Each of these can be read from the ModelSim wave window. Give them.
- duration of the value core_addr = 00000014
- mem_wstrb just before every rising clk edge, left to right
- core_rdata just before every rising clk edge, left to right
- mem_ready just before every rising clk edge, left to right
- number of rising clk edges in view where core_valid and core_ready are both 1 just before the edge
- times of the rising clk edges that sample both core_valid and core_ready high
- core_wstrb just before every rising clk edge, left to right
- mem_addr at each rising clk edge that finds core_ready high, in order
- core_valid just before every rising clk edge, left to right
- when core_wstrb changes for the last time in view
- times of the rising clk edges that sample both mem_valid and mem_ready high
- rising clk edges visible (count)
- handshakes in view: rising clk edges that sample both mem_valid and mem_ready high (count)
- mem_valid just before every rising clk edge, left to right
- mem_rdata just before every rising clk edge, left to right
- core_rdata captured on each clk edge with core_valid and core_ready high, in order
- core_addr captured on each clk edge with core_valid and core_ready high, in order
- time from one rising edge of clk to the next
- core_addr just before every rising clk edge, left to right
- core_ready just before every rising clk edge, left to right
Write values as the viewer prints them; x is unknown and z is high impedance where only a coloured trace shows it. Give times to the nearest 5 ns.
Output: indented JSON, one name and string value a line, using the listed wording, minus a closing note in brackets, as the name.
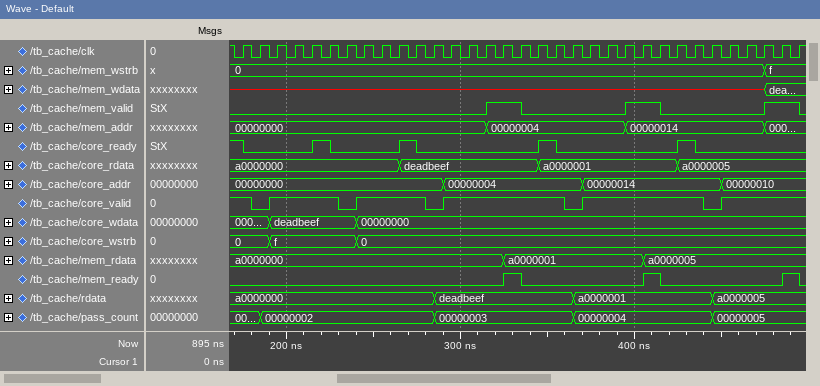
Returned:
{
  "duration of the value core_addr = 00000014": "80 ns",
  "mem_wstrb just before every rising clk edge, left to right": "0, 0, 0, 0, 0, 0, 0, 0, 0, 0, 0, 0, 0, 0, 0, 0, 0, 0, 0, 0, 0, 0, 0, 0, 0, 0, 0, 0, 0, 0, 0, f, f",
  "core_rdata just before every rising clk edge, left to right": "a0000000, a0000000, a0000000, a0000000, a0000000, a0000000, a0000000, a0000000, a0000000, a0000000, deadbeef, deadbeef, deadbeef, deadbeef, deadbeef, deadbeef, deadbeef, deadbeef, a0000001, a0000001, a0000001, a0000001, a0000001, a0000001, a0000001, a0000001, a0000005, a0000005, a0000005, a0000005, a0000005, a0000005, a0000005",
  "mem_ready just before every rising clk edge, left to right": "0 0 0 0 0 0 0 0 0 0 0 0 0 0 0 0 1 0 0 0 0 0 0 0 1 0 0 0 0 0 0 0 1",
  "number of rising clk edges in view where core_valid and core_ready are both 1 just before the edge": "5",
  "times of the rising clk edges that sample both core_valid and core_ready high": "175 ns, 225 ns, 275 ns, 355 ns, 435 ns",
  "core_wstrb just before every rising clk edge, left to right": "0, 0, f, f, f, f, f, 0, 0, 0, 0, 0, 0, 0, 0, 0, 0, 0, 0, 0, 0, 0, 0, 0, 0, 0, 0, 0, 0, 0, 0, 0, 0",
  "mem_addr at each rising clk edge that finds core_ready high, in order": "00000000, 00000000, 00000000, 00000004, 00000014",
  "core_valid just before every rising clk edge, left to right": "1 0 1 1 1 1 0 1 1 1 1 0 1 1 1 1 1 1 1 0 1 1 1 1 1 1 1 0 1 1 1 1 1",
  "when core_wstrb changes for the last time in view": "240 ns",
  "times of the rising clk edges that sample both mem_valid and mem_ready high": "335 ns, 415 ns, 495 ns",
  "rising clk edges visible": "33",
  "handshakes in view: rising clk edges that sample both mem_valid and mem_ready high": "3",
  "mem_valid just before every rising clk edge, left to right": "0 0 0 0 0 0 0 0 0 0 0 0 0 0 0 1 1 0 0 0 0 0 0 1 1 0 0 0 0 0 0 1 1",
  "mem_rdata just before every rising clk edge, left to right": "a0000000, a0000000, a0000000, a0000000, a0000000, a0000000, a0000000, a0000000, a0000000, a0000000, a0000000, a0000000, a0000000, a0000000, a0000000, a0000000, a0000001, a0000001, a0000001, a0000001, a0000001, a0000001, a0000001, a0000001, a0000005, a0000005, a0000005, a0000005, a0000005, a0000005, a0000005, a0000005, a0000005",
  "core_rdata captured on each clk edge with core_valid and core_ready high, in order": "a0000000, a0000000, deadbeef, a0000001, a0000005",
  "core_addr captured on each clk edge with core_valid and core_ready high, in order": "00000000, 00000000, 00000000, 00000004, 00000014",
  "time from one rising edge of clk to the next": "10 ns",
  "core_addr just before every rising clk edge, left to right": "00000000, 00000000, 00000000, 00000000, 00000000, 00000000, 00000000, 00000000, 00000000, 00000000, 00000000, 00000000, 00000004, 00000004, 00000004, 00000004, 00000004, 00000004, 00000004, 00000004, 00000014, 00000014, 00000014, 00000014, 00000014, 00000014, 00000014, 00000014, 00000010, 00000010, 00000010, 00000010, 00000010",
  "core_ready just before every rising clk edge, left to right": "1 0 0 0 0 1 0 0 0 0 1 0 0 0 0 0 0 0 1 0 0 0 0 0 0 0 1 0 0 0 0 0 0"
}
